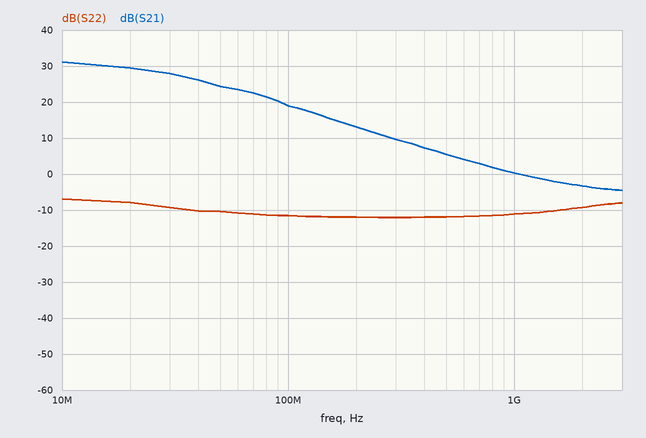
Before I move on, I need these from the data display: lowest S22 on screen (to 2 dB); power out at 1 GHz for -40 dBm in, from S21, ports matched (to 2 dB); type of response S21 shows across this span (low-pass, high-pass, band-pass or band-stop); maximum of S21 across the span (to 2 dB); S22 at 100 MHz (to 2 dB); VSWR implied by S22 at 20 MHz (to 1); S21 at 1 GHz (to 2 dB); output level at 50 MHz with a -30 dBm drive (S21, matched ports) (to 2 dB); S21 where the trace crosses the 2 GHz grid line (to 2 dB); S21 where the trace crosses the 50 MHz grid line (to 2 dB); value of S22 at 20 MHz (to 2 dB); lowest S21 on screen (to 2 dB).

-12 dB
-40 dBm
low-pass
32 dB
-12 dB
2
0 dB
-6 dBm
-4 dB
24 dB
-8 dB
-4 dB
